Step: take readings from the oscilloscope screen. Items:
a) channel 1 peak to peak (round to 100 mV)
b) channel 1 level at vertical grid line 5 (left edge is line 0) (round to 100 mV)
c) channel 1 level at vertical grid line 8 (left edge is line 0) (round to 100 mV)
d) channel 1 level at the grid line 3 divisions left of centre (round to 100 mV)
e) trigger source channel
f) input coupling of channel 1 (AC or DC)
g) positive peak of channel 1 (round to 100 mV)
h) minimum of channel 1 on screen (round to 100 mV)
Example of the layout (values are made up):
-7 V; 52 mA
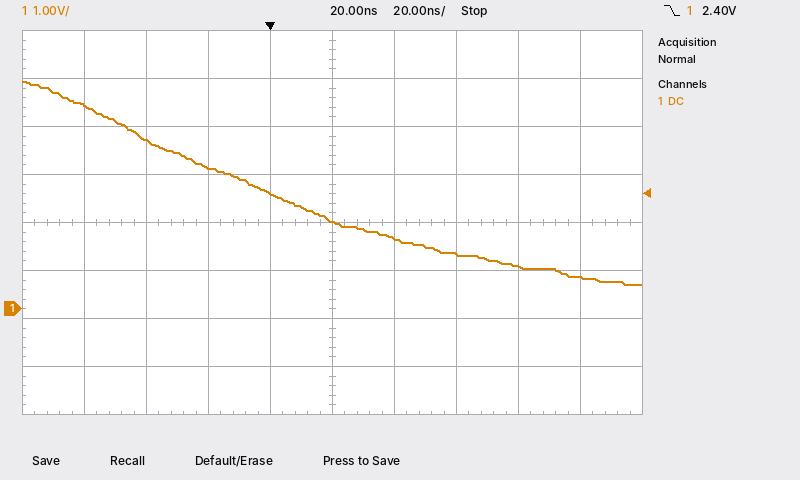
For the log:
4.2 V; 1.8 V; 900 mV; 3.5 V; channel 1; DC; 4.7 V; 500 mV
